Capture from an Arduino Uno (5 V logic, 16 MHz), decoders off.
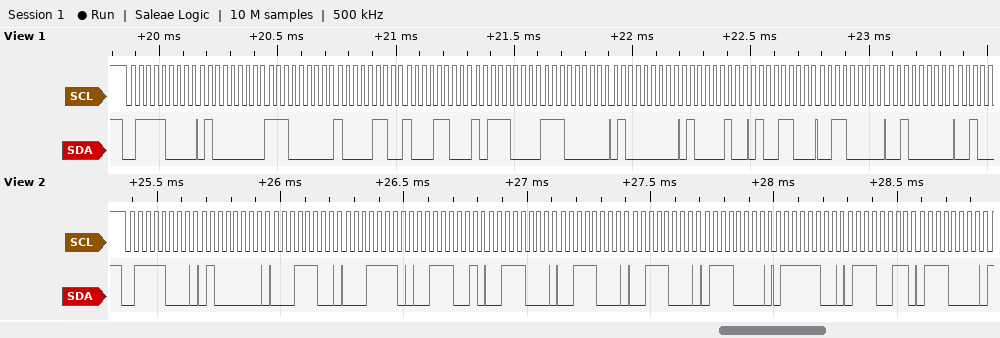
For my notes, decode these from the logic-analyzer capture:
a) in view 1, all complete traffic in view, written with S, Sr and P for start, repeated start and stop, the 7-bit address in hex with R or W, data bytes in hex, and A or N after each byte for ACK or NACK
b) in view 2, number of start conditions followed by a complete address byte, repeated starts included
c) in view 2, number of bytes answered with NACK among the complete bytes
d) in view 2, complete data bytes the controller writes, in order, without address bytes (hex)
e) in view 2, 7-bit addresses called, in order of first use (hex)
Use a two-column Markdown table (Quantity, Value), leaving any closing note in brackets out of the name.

| Quantity | Value |
|---|---|
| in view 1, all complete traffic in view, written with S, Sr and P for start, repeated start and stop, the 7-bit address in hex with R or W, data bytes in hex, and A or N after each byte for ACK or NACK | S 3CW A 40 A E0 A 86 A 8C A B8 A E0 A 40 A 42 A 4C A 30 A 20 A |
| in view 2, number of start conditions followed by a complete address byte, repeated starts included | 1 |
| in view 2, number of bytes answered with NACK among the complete bytes | 0 |
| in view 2, complete data bytes the controller writes, in order, without address bytes | 40 1C 1E 39 38 38 38 70 7C 73 70 |
| in view 2, 7-bit addresses called, in order of first use | 0x3C |
